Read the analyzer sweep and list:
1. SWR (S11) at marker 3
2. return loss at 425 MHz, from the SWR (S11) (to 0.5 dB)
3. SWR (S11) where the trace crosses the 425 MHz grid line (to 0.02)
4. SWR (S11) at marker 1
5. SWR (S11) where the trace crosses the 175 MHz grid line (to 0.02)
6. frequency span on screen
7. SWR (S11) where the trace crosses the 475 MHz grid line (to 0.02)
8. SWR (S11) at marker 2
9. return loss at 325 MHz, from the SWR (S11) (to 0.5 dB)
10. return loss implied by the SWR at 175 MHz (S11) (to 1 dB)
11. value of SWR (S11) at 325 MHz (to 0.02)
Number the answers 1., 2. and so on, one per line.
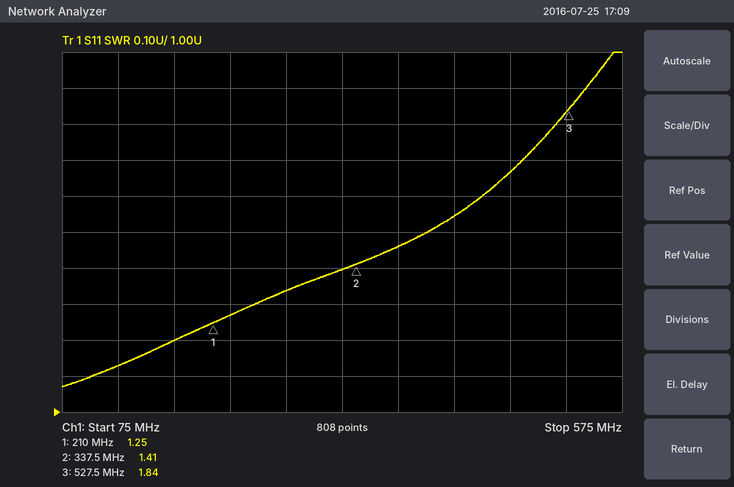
1. 1.84
2. 13.5 dB
3. 1.54
4. 1.25
5. 1.20
6. 500 MHz
7. 1.66
8. 1.41
9. 15.5 dB
10. 21 dB
11. 1.40
